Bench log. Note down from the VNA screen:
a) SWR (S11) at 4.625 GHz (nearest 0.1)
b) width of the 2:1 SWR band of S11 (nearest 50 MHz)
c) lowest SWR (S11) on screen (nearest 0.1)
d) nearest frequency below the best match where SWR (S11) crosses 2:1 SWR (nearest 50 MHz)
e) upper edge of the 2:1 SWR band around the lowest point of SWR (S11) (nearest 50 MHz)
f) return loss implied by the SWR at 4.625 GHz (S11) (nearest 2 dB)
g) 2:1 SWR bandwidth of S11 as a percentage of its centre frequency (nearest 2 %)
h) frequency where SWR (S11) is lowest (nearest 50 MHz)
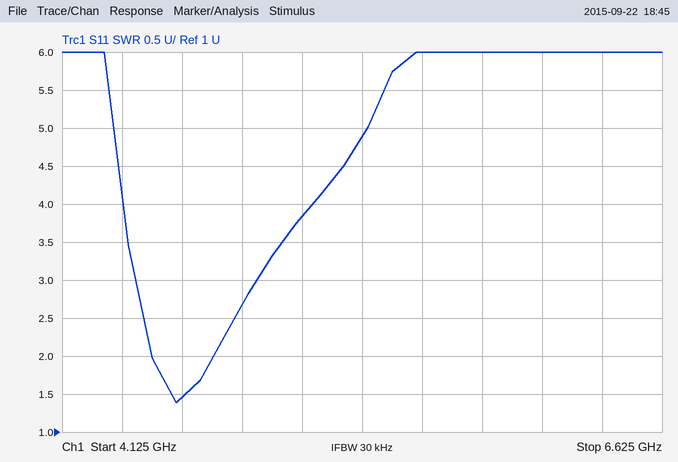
1.5
250 MHz
1.4
4.50 GHz
4.75 GHz
14 dB
6 %
4.60 GHz
